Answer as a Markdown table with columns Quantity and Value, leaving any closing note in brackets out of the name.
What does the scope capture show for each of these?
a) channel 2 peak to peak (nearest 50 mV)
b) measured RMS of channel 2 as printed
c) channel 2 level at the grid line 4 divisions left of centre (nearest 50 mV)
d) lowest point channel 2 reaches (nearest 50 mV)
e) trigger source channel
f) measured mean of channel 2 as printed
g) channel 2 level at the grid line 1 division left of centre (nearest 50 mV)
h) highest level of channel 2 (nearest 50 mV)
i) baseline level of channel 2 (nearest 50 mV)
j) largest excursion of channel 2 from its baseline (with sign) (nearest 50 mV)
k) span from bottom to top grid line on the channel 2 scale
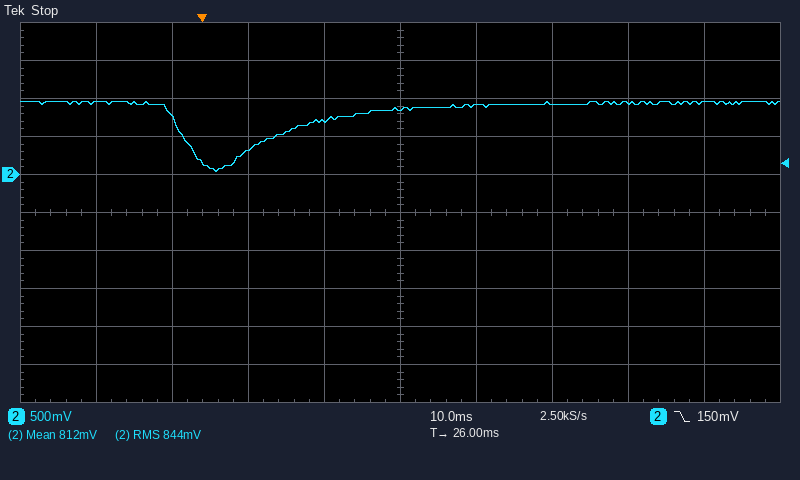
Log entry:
| Quantity | Value |
|---|---|
| channel 2 peak to peak | 900 mV |
| measured RMS of channel 2 as printed | 844 mV |
| channel 2 level at the grid line 4 divisions left of centre | 950 mV |
| lowest point channel 2 reaches | 50 mV |
| trigger source channel | channel 2 |
| measured mean of channel 2 as printed | 812 mV |
| channel 2 level at the grid line 1 division left of centre | 700 mV |
| highest level of channel 2 | 950 mV |
| baseline level of channel 2 | 950 mV |
| largest excursion of channel 2 from its baseline (with sign) | -900 mV |
| span from bottom to top grid line on the channel 2 scale | 5 V |
